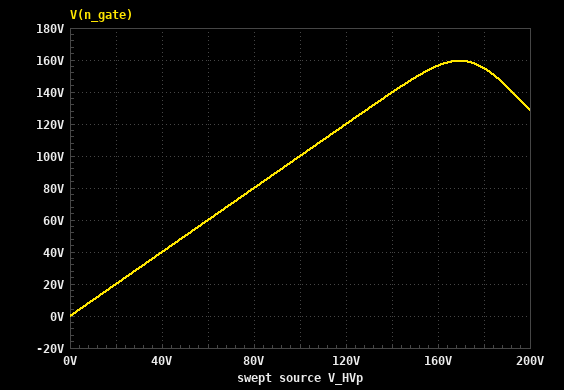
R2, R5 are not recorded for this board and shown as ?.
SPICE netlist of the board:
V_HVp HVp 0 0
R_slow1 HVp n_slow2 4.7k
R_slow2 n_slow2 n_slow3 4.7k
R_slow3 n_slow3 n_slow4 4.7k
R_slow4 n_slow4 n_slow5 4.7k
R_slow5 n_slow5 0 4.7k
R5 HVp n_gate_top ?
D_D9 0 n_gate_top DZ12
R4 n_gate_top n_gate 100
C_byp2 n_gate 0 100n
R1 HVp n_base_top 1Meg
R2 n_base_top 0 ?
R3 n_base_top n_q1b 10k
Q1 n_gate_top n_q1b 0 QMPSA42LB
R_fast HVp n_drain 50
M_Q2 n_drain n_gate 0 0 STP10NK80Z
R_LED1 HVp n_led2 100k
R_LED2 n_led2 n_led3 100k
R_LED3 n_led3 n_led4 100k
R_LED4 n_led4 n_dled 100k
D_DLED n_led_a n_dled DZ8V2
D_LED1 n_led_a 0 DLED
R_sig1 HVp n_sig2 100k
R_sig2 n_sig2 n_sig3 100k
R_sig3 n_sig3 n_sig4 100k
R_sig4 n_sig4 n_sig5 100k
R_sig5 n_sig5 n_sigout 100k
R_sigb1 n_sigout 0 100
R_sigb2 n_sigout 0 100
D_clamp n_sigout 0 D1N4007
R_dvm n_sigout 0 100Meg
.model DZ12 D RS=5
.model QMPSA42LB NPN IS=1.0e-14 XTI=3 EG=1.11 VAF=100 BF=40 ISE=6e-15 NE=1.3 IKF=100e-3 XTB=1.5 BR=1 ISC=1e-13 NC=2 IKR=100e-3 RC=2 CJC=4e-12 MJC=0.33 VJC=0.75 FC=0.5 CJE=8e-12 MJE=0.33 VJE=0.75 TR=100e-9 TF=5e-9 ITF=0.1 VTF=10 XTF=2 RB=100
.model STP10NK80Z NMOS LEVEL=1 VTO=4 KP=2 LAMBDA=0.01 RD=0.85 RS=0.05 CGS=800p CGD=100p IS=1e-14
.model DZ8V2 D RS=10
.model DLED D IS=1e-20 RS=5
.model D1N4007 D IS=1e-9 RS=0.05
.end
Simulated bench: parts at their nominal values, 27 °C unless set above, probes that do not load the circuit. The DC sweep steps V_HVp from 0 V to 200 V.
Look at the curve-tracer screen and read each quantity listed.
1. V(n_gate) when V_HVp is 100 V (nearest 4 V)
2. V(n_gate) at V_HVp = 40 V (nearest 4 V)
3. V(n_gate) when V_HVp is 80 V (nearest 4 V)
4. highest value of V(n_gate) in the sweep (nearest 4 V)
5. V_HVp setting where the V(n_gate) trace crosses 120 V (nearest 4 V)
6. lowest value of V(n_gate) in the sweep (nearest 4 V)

100 V
40 V
80 V
160 V
120 V
0 V
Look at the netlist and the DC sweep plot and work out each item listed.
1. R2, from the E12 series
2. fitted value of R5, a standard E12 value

3.3 kΩ
220 kΩ
